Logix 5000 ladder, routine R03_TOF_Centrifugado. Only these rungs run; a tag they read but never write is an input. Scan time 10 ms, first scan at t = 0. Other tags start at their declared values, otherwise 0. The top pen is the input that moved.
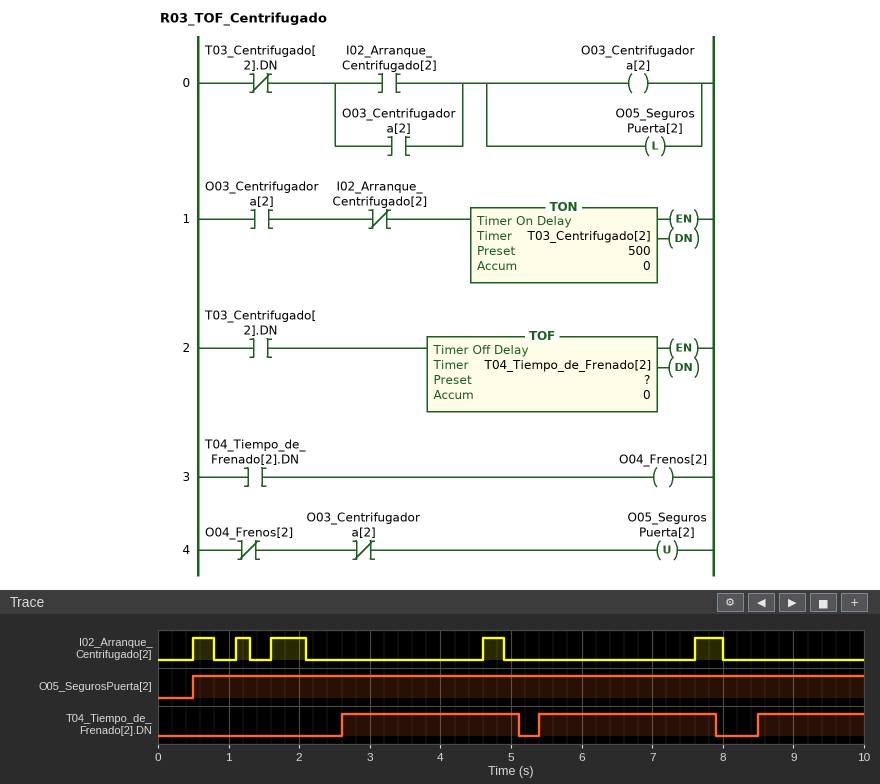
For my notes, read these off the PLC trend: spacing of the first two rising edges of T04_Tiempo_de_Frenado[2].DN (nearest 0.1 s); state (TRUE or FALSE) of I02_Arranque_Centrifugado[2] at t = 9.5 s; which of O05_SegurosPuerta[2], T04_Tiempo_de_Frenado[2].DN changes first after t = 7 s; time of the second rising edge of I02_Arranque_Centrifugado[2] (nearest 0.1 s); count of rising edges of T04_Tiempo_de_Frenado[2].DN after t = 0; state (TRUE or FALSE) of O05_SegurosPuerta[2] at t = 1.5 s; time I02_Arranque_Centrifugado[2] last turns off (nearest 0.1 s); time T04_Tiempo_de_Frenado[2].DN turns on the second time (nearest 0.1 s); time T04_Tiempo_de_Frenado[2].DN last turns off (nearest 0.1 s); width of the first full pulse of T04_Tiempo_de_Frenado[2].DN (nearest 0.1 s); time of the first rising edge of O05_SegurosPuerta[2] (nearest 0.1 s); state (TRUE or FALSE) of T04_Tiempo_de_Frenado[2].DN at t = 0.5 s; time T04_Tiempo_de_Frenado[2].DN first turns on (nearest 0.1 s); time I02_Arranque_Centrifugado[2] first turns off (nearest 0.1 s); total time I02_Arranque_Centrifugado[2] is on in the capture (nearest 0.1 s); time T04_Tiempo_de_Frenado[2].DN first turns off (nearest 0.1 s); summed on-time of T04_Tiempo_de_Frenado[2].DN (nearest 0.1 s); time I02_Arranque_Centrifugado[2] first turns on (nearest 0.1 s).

2.8 s
FALSE
T04_Tiempo_de_Frenado[2].DN
1.1 s
3
TRUE
8.0 s
5.4 s
7.9 s
2.5 s
0.5 s
FALSE
2.6 s
0.8 s
1.7 s
5.1 s
6.5 s
0.5 s
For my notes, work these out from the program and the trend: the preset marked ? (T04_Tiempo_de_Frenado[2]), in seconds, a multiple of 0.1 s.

2.5 s
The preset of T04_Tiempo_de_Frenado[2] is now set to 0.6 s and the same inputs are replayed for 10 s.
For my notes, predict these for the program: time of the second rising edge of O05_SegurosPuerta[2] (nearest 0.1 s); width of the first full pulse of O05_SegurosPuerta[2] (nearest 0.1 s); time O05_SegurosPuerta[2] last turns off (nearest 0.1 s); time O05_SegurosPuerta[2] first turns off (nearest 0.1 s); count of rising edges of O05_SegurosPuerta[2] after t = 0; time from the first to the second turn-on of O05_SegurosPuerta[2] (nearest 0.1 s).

4.6 s
2.7 s
9.1 s
3.2 s
3
4.1 s
